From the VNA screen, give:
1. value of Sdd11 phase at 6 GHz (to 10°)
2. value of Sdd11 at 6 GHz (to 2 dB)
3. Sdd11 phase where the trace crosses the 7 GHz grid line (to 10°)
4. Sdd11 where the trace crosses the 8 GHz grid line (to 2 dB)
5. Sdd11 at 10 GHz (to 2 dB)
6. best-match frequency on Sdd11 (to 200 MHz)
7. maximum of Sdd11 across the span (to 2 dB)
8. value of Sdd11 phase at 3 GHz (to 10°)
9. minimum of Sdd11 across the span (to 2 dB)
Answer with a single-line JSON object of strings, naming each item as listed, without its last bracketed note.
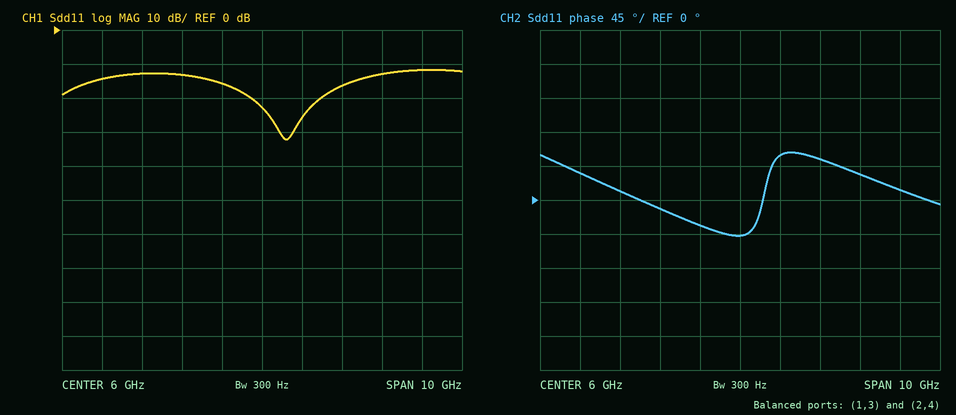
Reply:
{"value of Sdd11 phase at 6 GHz": "-50°", "value of Sdd11 at 6 GHz": "-22 dB", "Sdd11 phase where the trace crosses the 7 GHz grid line": "60°", "Sdd11 where the trace crosses the 8 GHz grid line": "-16 dB", "Sdd11 at 10 GHz": "-12 dB", "best-match frequency on Sdd11": "6.6 GHz", "maximum of Sdd11 across the span": "-12 dB", "value of Sdd11 phase at 3 GHz": "10°", "minimum of Sdd11 across the span": "-32 dB"}
